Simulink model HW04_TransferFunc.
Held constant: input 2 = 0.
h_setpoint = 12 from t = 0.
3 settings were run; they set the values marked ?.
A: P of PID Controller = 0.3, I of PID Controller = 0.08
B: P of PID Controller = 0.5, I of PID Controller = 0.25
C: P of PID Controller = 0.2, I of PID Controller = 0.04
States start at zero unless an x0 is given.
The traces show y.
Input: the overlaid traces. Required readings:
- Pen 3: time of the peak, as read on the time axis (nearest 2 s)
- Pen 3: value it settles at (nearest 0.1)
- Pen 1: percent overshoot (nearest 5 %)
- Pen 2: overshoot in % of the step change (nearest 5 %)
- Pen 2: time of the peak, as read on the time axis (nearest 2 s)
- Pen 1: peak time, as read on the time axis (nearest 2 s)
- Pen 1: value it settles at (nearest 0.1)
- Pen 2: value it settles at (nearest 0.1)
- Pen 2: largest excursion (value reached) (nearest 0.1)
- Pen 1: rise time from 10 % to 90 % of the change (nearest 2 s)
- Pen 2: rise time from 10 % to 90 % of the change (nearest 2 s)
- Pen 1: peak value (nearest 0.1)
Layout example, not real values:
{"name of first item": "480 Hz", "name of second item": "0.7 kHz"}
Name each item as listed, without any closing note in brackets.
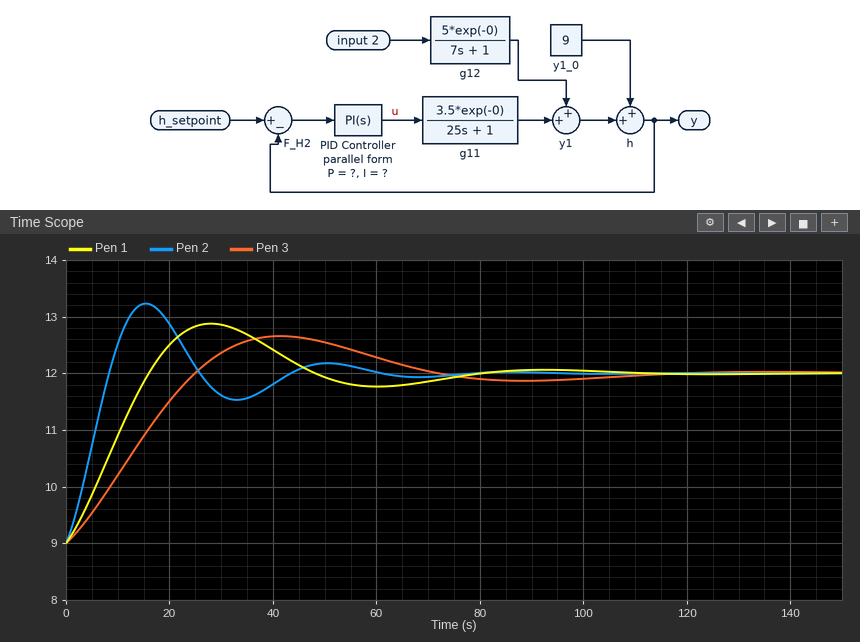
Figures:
{"Pen 3: time of the peak, as read on the time axis": "42 s", "Pen 3: value it settles at": "12.0", "Pen 1: percent overshoot": "30 %", "Pen 2: overshoot in % of the step change": "40 %", "Pen 2: time of the peak, as read on the time axis": "16 s", "Pen 1: peak time, as read on the time axis": "28 s", "Pen 1: value it settles at": "12.0", "Pen 2: value it settles at": "12.0", "Pen 2: largest excursion (value reached)": "13.2", "Pen 1: rise time from 10 % to 90 % of the change": "12 s", "Pen 2: rise time from 10 % to 90 % of the change": "6 s", "Pen 1: peak value": "12.9"}
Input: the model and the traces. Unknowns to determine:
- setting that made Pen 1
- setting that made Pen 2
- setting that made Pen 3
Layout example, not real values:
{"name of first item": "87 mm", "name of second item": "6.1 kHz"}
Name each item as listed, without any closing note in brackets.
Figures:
{"setting that made Pen 1": "A", "setting that made Pen 2": "B", "setting that made Pen 3": "C"}
